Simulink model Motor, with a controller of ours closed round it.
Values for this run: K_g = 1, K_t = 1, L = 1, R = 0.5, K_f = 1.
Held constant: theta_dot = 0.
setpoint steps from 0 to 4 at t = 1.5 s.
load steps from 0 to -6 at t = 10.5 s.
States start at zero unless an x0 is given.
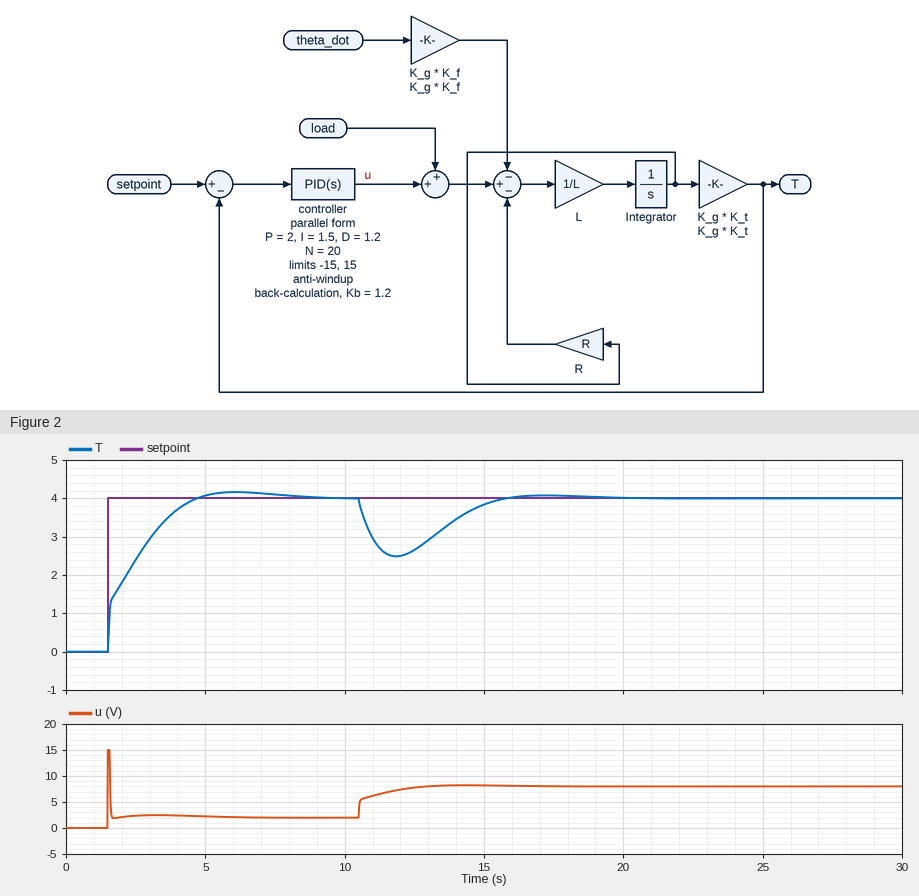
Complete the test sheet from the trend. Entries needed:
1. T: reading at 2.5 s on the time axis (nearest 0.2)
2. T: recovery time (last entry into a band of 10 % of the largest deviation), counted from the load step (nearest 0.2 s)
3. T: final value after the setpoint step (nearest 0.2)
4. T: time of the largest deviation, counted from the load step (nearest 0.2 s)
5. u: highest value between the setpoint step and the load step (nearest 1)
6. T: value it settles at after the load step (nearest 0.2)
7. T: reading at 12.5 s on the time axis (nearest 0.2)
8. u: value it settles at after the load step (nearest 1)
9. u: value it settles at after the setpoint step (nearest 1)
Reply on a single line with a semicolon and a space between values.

2.4; 4.6 s; 4.0; 1.4 s; 15; 4.0; 2.6; 8; 2
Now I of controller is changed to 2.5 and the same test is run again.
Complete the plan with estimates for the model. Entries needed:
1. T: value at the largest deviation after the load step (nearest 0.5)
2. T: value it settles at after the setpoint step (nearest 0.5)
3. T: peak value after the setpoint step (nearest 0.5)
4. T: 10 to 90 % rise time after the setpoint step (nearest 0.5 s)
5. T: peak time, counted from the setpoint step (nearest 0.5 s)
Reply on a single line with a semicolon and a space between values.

2.5; 4.0; 4.5; 1.5 s; 3.0 s
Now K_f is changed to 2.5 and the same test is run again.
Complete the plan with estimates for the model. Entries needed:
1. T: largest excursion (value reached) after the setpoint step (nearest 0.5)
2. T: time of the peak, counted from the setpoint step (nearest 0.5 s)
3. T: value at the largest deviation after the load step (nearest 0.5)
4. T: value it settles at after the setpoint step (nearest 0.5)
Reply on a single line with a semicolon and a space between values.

4.0; 4.5 s; 2.5; 4.0
